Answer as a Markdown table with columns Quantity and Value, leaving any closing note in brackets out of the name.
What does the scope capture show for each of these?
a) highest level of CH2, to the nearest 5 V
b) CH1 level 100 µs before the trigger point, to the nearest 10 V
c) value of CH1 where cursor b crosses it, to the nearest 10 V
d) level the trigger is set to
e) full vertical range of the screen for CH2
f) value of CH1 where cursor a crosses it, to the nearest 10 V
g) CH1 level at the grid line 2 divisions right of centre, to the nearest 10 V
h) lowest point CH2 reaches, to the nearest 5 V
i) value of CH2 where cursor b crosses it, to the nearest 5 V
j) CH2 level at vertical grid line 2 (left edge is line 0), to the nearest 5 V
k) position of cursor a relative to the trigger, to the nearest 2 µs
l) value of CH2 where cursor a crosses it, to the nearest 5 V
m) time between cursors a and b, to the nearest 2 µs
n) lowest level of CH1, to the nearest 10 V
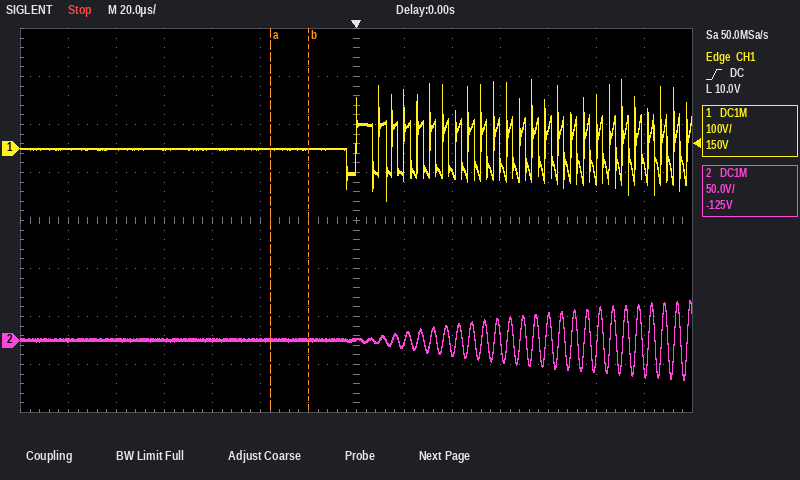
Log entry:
| Quantity | Value |
|---|---|
| highest level of CH2, to the nearest 5 V | 40 V |
| CH1 level 100 µs before the trigger point, to the nearest 10 V | 0 V |
| value of CH1 where cursor b crosses it, to the nearest 10 V | 0 V |
| level the trigger is set to | 10.0 V |
| full vertical range of the screen for CH2 | 400 V |
| value of CH1 where cursor a crosses it, to the nearest 10 V | 0 V |
| CH1 level at the grid line 2 divisions right of centre, to the nearest 10 V | -50 V |
| lowest point CH2 reaches, to the nearest 5 V | -40 V |
| value of CH2 where cursor b crosses it, to the nearest 5 V | 0 V |
| CH2 level at vertical grid line 2 (left edge is line 0), to the nearest 5 V | 0 V |
| position of cursor a relative to the trigger, to the nearest 2 µs | -36 µs |
| value of CH2 where cursor a crosses it, to the nearest 5 V | 0 V |
| time between cursors a and b, to the nearest 2 µs | 16 µs |
| lowest level of CH1, to the nearest 10 V | -110 V |
